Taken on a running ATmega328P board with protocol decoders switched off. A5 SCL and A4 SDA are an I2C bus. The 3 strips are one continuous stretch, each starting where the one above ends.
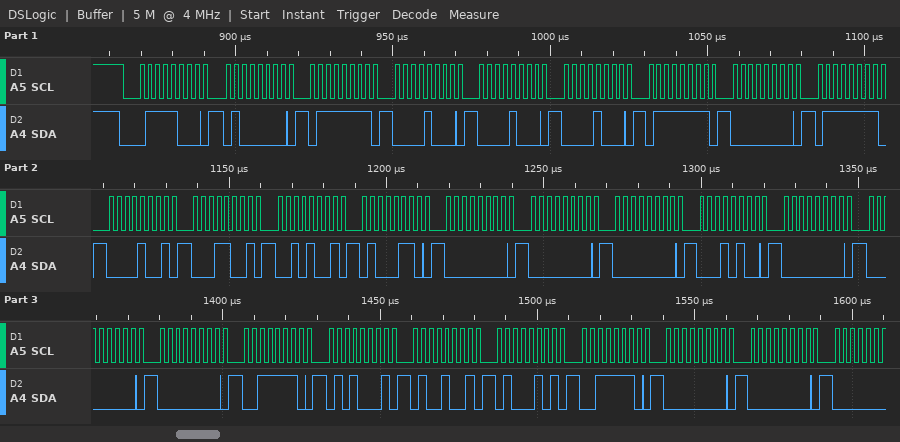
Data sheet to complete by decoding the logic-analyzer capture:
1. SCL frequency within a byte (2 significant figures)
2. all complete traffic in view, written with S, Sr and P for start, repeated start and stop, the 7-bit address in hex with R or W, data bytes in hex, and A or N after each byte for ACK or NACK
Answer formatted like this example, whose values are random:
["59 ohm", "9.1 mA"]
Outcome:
["400 kHz", "S 3CW A 40 A 7F A 08 A 08 A 08 A 7F A 00 A 7F A 09 A 19 A 29 A 46 A 00 A 00 A 00 A 14 A 00 A 00 A 00 A 3E A 51 A 49 A 45 A 3E A 00 A 00 A"]
